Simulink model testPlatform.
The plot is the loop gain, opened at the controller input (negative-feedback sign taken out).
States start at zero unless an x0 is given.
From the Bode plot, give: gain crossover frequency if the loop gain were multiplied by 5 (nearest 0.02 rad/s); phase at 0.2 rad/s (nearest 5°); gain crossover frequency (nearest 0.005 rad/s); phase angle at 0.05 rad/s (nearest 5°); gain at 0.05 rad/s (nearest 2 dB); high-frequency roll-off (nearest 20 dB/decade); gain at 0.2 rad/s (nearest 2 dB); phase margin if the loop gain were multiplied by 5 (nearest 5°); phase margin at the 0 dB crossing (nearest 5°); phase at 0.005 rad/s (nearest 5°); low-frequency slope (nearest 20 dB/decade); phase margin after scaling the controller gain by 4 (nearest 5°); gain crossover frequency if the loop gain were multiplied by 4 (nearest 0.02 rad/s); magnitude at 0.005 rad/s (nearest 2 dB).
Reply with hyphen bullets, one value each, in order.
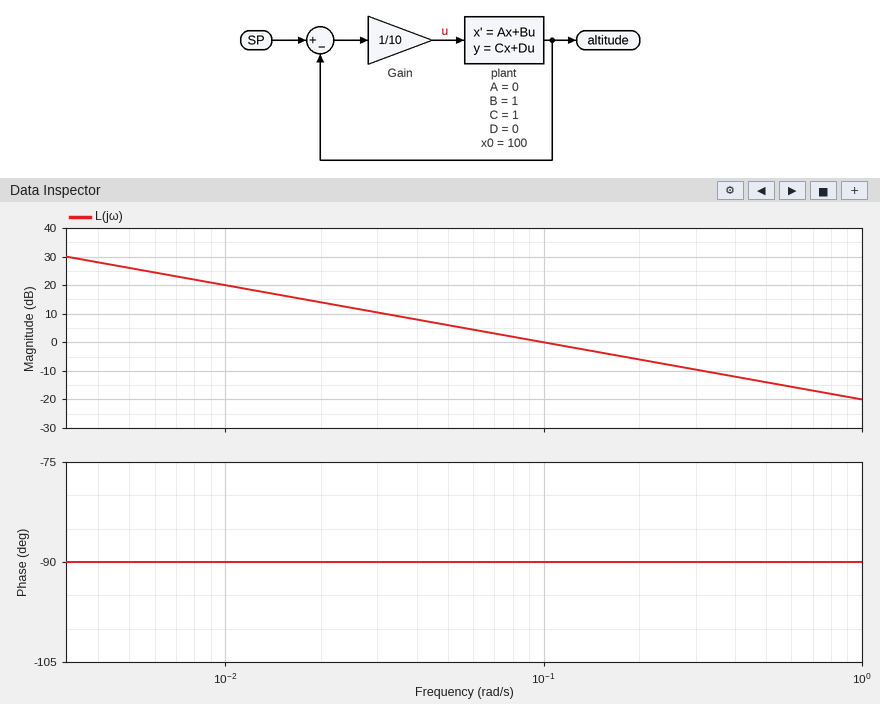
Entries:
- 0.50 rad/s
- -90°
- 0.100 rad/s
- -90°
- 6 dB
- -20 dB/decade
- -6 dB
- 90°
- 90°
- -90°
- -20 dB/decade
- 90°
- 0.40 rad/s
- 26 dB
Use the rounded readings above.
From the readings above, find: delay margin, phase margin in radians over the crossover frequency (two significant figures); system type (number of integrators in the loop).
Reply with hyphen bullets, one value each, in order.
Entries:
- 16 s
- 1
